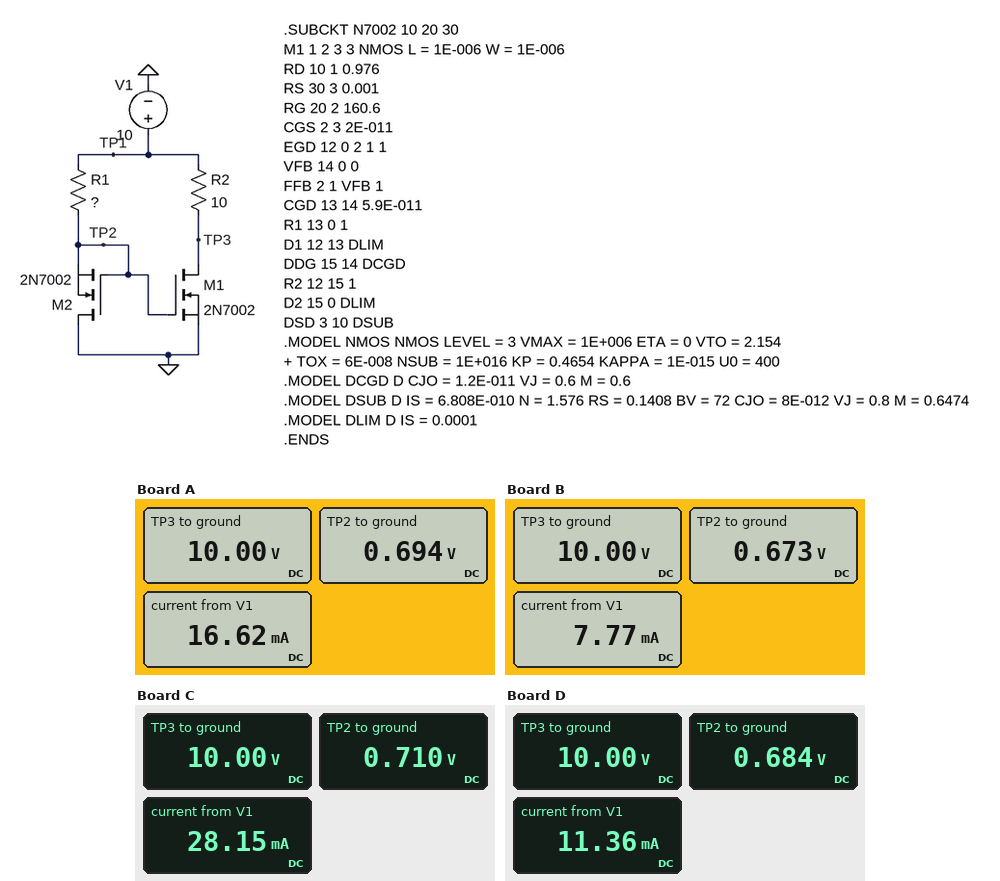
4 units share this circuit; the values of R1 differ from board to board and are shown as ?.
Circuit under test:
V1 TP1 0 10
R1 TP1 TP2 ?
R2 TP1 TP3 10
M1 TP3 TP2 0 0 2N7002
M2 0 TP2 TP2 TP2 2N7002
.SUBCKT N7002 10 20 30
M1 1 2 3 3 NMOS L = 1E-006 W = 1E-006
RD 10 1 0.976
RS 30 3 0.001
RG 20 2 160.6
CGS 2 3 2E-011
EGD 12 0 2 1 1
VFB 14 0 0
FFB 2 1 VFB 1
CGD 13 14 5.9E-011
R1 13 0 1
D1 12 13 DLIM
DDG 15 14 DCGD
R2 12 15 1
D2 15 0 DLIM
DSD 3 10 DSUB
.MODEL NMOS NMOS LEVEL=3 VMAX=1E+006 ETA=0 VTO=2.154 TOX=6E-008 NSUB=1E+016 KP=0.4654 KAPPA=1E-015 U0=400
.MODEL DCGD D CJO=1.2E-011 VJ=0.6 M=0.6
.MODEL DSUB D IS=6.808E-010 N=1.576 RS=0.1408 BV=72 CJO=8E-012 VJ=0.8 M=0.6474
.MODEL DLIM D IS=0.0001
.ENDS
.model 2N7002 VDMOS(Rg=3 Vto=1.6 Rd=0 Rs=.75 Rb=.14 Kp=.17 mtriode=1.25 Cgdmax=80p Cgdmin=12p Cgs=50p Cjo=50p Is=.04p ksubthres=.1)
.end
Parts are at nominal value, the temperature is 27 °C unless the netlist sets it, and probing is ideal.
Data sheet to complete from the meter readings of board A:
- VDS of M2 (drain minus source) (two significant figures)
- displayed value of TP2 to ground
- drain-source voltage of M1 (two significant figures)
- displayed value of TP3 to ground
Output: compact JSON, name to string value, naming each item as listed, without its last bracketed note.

{"VDS of M2 (drain minus source)": "-690 mV", "displayed value of TP2 to ground": "0.694 V", "drain-source voltage of M1": "10 V", "displayed value of TP3 to ground": "10.00 V"}
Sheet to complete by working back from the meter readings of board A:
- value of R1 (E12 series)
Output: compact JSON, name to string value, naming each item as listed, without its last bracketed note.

{"value of R1": "560 Ω"}
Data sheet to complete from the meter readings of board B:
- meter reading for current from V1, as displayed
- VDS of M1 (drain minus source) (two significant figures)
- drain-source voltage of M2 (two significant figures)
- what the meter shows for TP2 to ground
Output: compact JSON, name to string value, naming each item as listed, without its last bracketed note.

{"meter reading for current from V1, as displayed": "7.77 mA", "VDS of M1 (drain minus source)": "10 V", "drain-source voltage of M2": "-670 mV", "what the meter shows for TP2 to ground": "0.673 V"}
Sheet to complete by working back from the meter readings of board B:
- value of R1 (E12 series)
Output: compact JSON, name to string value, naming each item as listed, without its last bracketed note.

{"value of R1": "1.2 kΩ"}
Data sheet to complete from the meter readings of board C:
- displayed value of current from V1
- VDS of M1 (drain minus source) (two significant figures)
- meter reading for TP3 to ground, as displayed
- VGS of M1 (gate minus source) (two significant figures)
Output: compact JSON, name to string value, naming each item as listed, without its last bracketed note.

{"displayed value of current from V1": "28.15 mA", "VDS of M1 (drain minus source)": "10 V", "meter reading for TP3 to ground, as displayed": "10.00 V", "VGS of M1 (gate minus source)": "710 mV"}
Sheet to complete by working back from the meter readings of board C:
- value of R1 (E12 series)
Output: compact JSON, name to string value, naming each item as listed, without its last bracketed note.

{"value of R1": "330 Ω"}
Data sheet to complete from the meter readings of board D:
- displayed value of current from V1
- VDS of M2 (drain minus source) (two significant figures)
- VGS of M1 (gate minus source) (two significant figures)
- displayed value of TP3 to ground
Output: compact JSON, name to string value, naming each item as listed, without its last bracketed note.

{"displayed value of current from V1": "11.36 mA", "VDS of M2 (drain minus source)": "-680 mV", "VGS of M1 (gate minus source)": "680 mV", "displayed value of TP3 to ground": "10.00 V"}
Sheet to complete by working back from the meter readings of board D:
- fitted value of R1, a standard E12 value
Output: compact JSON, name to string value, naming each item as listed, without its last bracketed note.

{"fitted value of R1, a standard E12 value": "820 Ω"}
